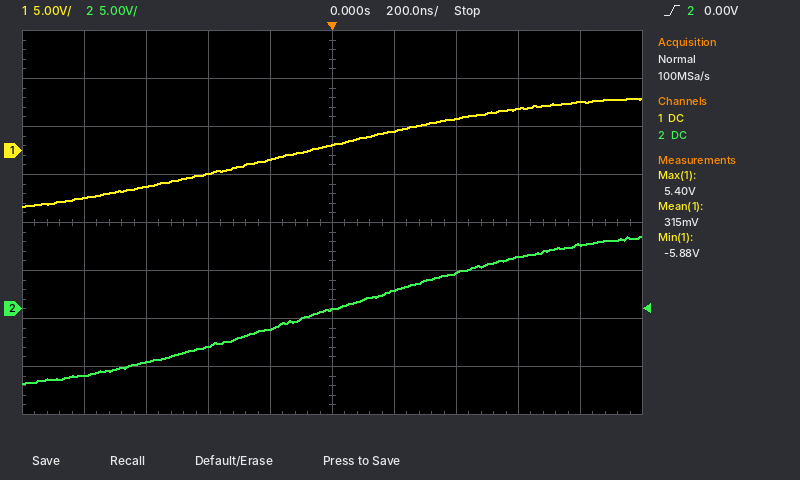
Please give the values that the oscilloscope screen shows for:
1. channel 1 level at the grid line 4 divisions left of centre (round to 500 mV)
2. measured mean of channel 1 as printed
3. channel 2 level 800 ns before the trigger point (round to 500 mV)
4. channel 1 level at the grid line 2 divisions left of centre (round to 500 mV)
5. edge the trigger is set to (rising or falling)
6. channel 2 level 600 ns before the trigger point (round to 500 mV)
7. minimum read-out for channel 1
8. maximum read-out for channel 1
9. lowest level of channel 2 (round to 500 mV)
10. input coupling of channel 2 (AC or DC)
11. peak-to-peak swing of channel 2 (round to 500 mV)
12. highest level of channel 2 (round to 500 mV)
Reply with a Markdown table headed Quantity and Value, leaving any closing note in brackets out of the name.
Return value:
| Quantity | Value |
|---|---|
| channel 1 level at the grid line 4 divisions left of centre | -5.0 V |
| measured mean of channel 1 as printed | 315 mV |
| channel 2 level 800 ns before the trigger point | -7.0 V |
| channel 1 level at the grid line 2 divisions left of centre | -2.5 V |
| edge the trigger is set to | rising |
| channel 2 level 600 ns before the trigger point | -5.5 V |
| minimum read-out for channel 1 | -5.88 V |
| maximum read-out for channel 1 | 5.40 V |
| lowest level of channel 2 | -8.0 V |
| input coupling of channel 2 | DC |
| peak-to-peak swing of channel 2 | 15.5 V |
| highest level of channel 2 | 7.5 V |
